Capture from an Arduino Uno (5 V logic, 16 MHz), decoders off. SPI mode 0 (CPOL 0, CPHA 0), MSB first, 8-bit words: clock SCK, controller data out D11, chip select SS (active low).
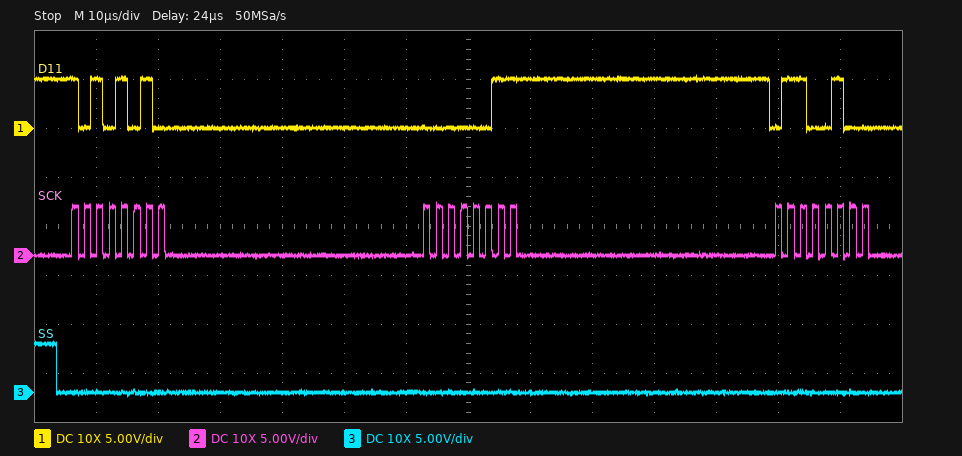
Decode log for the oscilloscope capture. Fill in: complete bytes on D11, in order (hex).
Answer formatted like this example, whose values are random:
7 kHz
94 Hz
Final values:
AA 03 64
